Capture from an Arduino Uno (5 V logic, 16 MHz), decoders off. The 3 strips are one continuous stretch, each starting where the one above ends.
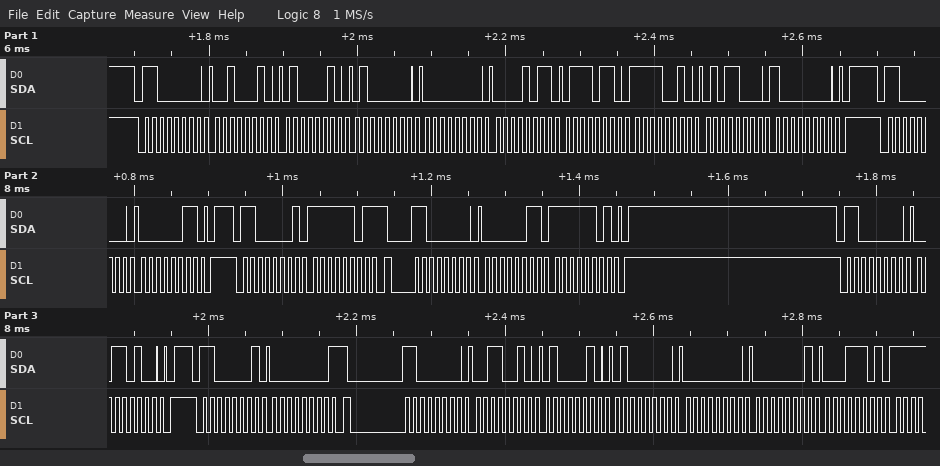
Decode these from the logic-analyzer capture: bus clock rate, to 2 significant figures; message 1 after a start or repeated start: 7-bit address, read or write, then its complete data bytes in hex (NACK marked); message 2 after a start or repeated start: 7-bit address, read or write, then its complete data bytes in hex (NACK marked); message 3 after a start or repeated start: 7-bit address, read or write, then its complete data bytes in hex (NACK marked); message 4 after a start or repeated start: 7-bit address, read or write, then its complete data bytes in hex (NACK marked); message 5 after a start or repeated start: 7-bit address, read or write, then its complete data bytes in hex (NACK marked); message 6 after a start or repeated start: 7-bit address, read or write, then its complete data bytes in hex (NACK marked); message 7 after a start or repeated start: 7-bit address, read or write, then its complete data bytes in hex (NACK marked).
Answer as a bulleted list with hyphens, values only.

- 100 kHz
- 0x60 write: 22 42 40 00 0B 76 F2 58 80
- 0x60 write: 03
- 0x60 read: FD NACK
- 0x60 write: 03 FD
- 0x60 write: 34
- 0x60 read: 00 NACK
- 0x60 write: 32 42 40 00 01 1D
